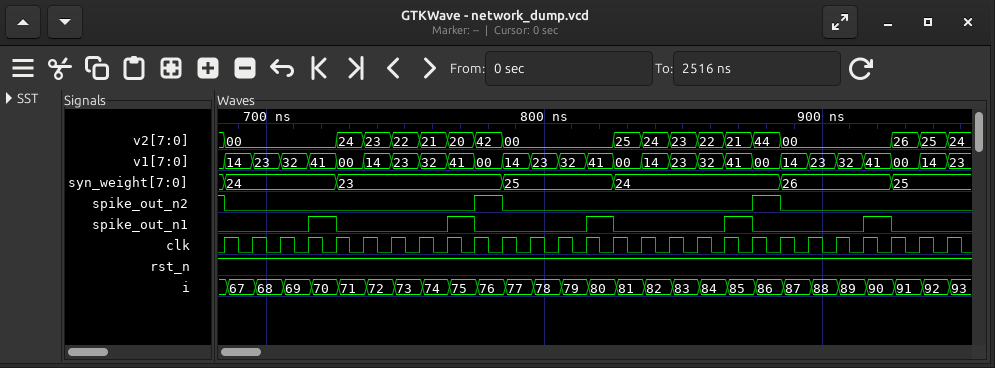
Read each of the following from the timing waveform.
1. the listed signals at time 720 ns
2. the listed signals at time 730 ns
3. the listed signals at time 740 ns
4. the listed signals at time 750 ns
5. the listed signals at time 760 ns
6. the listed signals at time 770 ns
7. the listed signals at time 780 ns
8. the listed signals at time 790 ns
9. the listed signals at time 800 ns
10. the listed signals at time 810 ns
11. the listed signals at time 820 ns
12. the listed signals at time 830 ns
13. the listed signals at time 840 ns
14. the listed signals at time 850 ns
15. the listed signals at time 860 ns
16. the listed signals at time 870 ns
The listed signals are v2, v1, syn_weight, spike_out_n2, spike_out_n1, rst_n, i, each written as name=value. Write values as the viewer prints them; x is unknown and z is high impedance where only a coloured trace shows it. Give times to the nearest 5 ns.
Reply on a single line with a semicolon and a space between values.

v2=00, v1=41, syn_weight=24, spike_out_n2=0, spike_out_n1=1, rst_n=1, i=70; v2=24, v1=00, syn_weight=23, spike_out_n2=0, spike_out_n1=0, rst_n=1, i=71; v2=23, v1=14, syn_weight=23, spike_out_n2=0, spike_out_n1=0, rst_n=1, i=72; v2=22, v1=23, syn_weight=23, spike_out_n2=0, spike_out_n1=0, rst_n=1, i=73; v2=21, v1=32, syn_weight=23, spike_out_n2=0, spike_out_n1=0, rst_n=1, i=74; v2=20, v1=41, syn_weight=23, spike_out_n2=0, spike_out_n1=1, rst_n=1, i=75; v2=42, v1=00, syn_weight=23, spike_out_n2=1, spike_out_n1=0, rst_n=1, i=76; v2=00, v1=14, syn_weight=25, spike_out_n2=0, spike_out_n1=0, rst_n=1, i=77; v2=00, v1=23, syn_weight=25, spike_out_n2=0, spike_out_n1=0, rst_n=1, i=78; v2=00, v1=32, syn_weight=25, spike_out_n2=0, spike_out_n1=0, rst_n=1, i=79; v2=00, v1=41, syn_weight=25, spike_out_n2=0, spike_out_n1=1, rst_n=1, i=80; v2=25, v1=00, syn_weight=24, spike_out_n2=0, spike_out_n1=0, rst_n=1, i=81; v2=24, v1=14, syn_weight=24, spike_out_n2=0, spike_out_n1=0, rst_n=1, i=82; v2=23, v1=23, syn_weight=24, spike_out_n2=0, spike_out_n1=0, rst_n=1, i=83; v2=22, v1=32, syn_weight=24, spike_out_n2=0, spike_out_n1=0, rst_n=1, i=84; v2=21, v1=41, syn_weight=24, spike_out_n2=0, spike_out_n1=1, rst_n=1, i=85
